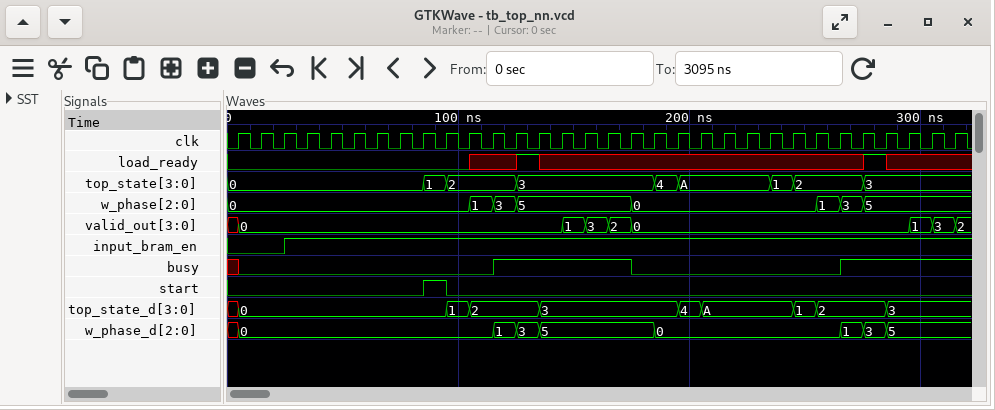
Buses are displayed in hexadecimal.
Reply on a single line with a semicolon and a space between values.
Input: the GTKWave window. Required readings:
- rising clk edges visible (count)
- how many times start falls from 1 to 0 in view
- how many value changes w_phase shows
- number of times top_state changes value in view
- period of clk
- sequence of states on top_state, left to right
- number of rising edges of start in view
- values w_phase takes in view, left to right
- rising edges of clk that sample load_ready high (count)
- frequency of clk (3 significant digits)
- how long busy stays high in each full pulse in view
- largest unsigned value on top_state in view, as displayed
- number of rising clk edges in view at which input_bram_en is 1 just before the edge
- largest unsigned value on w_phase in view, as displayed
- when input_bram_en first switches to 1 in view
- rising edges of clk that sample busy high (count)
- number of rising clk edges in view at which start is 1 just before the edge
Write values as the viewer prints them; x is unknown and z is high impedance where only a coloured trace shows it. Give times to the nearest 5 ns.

32; 1; 7; 8; 10 ns; 0, 1, 2, 3, 4, A, 1, 2, 3; 1; 0, 1, 3, 5, 0, 1, 3, 5; 2; 100 MHz; 60 ns; A; 29; 5; 25 ns; 11; 1
